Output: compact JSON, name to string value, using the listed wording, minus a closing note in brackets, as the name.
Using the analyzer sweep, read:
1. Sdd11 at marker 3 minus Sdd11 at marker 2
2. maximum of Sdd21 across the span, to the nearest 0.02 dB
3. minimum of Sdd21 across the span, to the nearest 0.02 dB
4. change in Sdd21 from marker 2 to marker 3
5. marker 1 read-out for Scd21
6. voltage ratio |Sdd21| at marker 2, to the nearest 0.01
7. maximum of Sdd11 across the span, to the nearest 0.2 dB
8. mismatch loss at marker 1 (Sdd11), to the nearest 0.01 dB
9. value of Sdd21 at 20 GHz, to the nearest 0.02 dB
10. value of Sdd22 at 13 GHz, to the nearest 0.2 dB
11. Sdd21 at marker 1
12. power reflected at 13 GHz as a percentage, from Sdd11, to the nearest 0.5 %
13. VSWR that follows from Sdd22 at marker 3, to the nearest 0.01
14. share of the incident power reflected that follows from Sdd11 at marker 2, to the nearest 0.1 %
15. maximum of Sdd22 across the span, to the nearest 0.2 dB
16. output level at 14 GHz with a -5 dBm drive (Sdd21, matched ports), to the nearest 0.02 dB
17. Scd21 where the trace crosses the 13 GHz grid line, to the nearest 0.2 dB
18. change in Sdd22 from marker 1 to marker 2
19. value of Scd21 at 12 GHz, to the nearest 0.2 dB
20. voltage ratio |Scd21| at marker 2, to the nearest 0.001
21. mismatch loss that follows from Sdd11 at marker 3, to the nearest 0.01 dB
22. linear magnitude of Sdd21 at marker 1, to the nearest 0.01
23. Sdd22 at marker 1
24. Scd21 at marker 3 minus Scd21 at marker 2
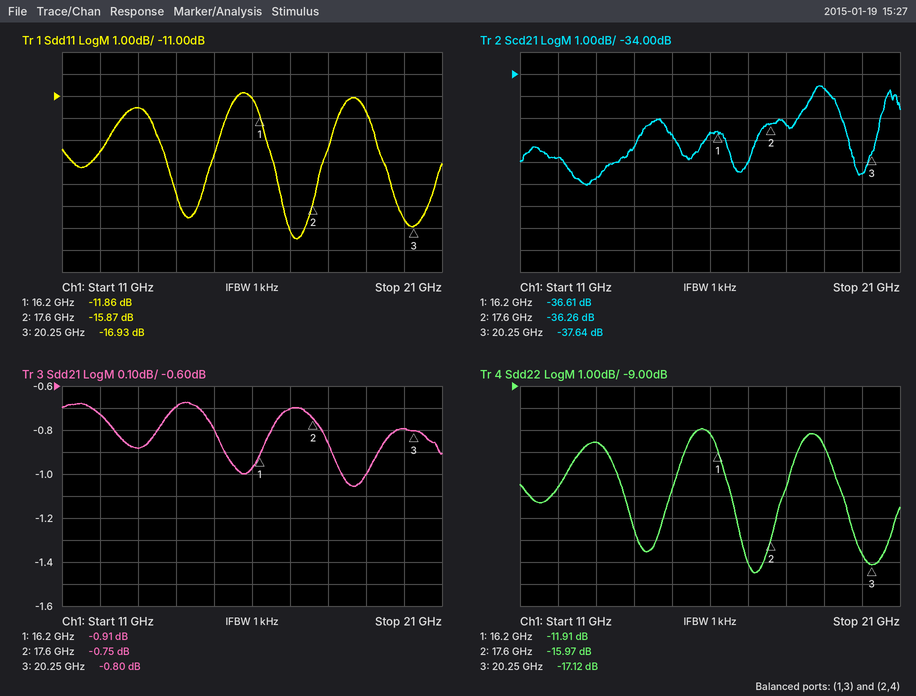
{"Sdd11 at marker 3 minus Sdd11 at marker 2": "-1.06 dB", "maximum of Sdd21 across the span, to the nearest 0.02 dB": "-0.68 dB", "minimum of Sdd21 across the span, to the nearest 0.02 dB": "-1.06 dB", "change in Sdd21 from marker 2 to marker 3": "-0.05 dB", "marker 1 read-out for Scd21": "-36.61 dB", "voltage ratio |Sdd21| at marker 2, to the nearest 0.01": "0.92", "maximum of Sdd11 across the span, to the nearest 0.2 dB": "-10.8 dB", "mismatch loss at marker 1 (Sdd11), to the nearest 0.01 dB": "0.29 dB", "value of Sdd21 at 20 GHz, to the nearest 0.02 dB": "-0.80 dB", "value of Sdd22 at 13 GHz, to the nearest 0.2 dB": "-11.6 dB", "Sdd21 at marker 1": "-0.91 dB", "power reflected at 13 GHz as a percentage, from Sdd11, to the nearest 0.5 %": "7.0 %", "VSWR that follows from Sdd22 at marker 3, to the nearest 0.01": "1.32", "share of the incident power reflected that follows from Sdd11 at marker 2, to the nearest 0.1 %": "2.6 %", "maximum of Sdd22 across the span, to the nearest 0.2 dB": "-11.0 dB", "output level at 14 GHz with a -5 dBm drive (Sdd21, matched ports), to the nearest 0.02 dB": "-5.70 dBm", "Scd21 where the trace crosses the 13 GHz grid line, to the nearest 0.2 dB": "-38.8 dB", "change in Sdd22 from marker 1 to marker 2": "-4.06 dB", "value of Scd21 at 12 GHz, to the nearest 0.2 dB": "-37.8 dB", "voltage ratio |Scd21| at marker 2, to the nearest 0.001": "0.015", "mismatch loss that follows from Sdd11 at marker 3, to the nearest 0.01 dB": "0.09 dB", "linear magnitude of Sdd21 at marker 1, to the nearest 0.01": "0.90", "Sdd22 at marker 1": "-11.91 dB", "Scd21 at marker 3 minus Scd21 at marker 2": "-1.38 dB"}
